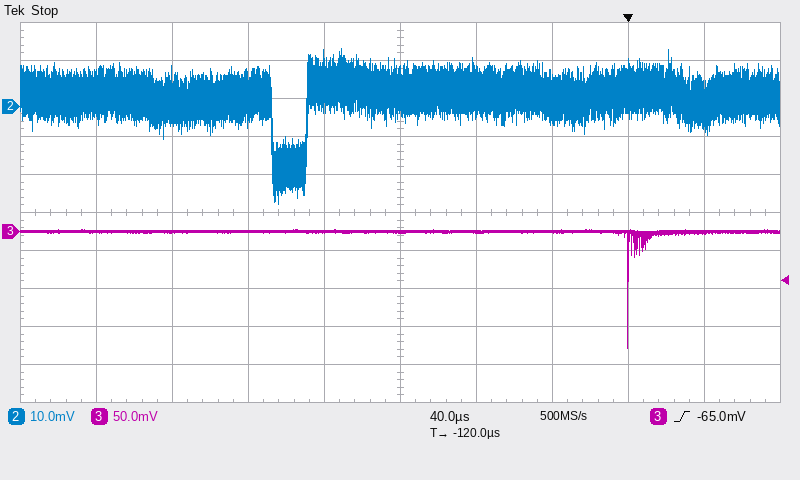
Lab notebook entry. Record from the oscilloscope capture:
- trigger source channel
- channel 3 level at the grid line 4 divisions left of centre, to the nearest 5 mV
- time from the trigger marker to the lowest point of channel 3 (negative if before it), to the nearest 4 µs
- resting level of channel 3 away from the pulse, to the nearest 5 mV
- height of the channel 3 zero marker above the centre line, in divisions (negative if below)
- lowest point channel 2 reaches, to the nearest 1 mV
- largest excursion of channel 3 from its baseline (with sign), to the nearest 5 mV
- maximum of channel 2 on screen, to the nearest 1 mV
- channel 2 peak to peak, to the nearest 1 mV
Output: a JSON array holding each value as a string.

["channel 3", "0 mV", "0 µs", "0 mV", "-0.5 div", "-26 mV", "-155 mV", "15 mV", "41 mV"]
